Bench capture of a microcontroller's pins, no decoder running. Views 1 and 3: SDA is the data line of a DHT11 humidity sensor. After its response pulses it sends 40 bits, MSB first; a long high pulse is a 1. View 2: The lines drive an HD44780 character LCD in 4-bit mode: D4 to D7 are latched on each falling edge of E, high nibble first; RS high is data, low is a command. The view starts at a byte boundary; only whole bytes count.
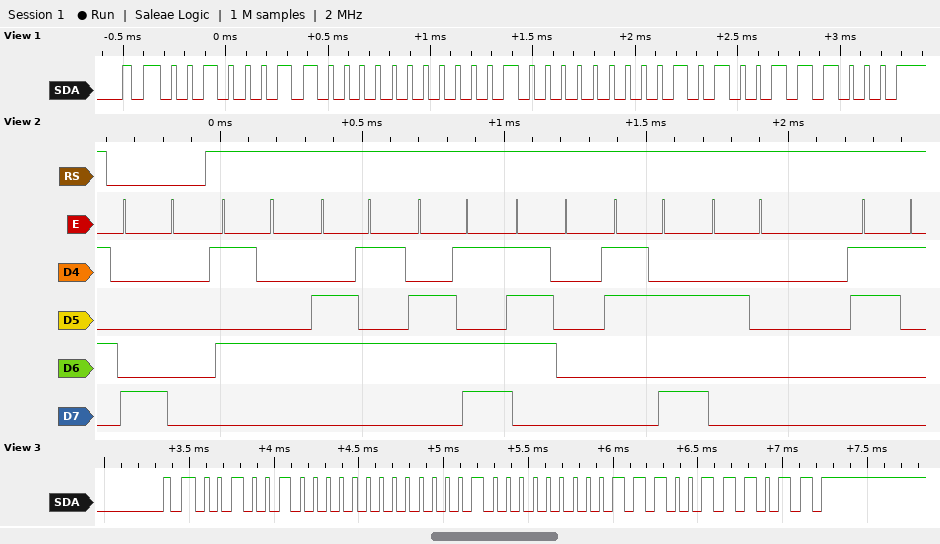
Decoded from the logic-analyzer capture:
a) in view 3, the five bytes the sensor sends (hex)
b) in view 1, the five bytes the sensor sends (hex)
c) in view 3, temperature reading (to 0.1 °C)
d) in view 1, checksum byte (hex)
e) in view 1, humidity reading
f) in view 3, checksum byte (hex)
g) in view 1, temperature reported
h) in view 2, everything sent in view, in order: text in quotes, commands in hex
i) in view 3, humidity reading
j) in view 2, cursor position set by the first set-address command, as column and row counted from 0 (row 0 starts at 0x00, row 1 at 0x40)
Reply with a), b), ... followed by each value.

a) 24 00 10 07 3B
b) 23 00 10 05 38
c) 16.7 °C
d) 0x38
e) 35 %
f) 0x3B
g) 16.5 °C
h) 0x80 "Temp: 1"
i) 36 %
j) column 0, row 0
